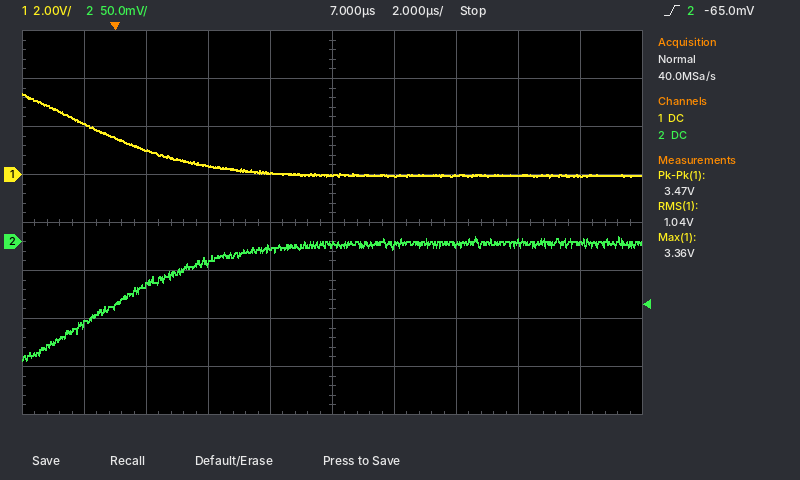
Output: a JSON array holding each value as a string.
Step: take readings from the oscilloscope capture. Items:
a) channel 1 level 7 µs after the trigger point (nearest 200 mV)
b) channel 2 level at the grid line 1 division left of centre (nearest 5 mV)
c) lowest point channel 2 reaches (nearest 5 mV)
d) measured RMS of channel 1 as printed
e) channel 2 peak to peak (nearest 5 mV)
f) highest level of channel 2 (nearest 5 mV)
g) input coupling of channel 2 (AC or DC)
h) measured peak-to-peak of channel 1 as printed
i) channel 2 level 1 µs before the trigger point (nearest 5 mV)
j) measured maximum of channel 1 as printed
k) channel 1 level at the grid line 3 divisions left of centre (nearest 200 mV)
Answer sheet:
["0.0 V", "-5 mV", "-125 mV", "1.04 V", "130 mV", "5 mV", "DC", "3.47 V", "-85 mV", "3.36 V", "1.0 V"]
